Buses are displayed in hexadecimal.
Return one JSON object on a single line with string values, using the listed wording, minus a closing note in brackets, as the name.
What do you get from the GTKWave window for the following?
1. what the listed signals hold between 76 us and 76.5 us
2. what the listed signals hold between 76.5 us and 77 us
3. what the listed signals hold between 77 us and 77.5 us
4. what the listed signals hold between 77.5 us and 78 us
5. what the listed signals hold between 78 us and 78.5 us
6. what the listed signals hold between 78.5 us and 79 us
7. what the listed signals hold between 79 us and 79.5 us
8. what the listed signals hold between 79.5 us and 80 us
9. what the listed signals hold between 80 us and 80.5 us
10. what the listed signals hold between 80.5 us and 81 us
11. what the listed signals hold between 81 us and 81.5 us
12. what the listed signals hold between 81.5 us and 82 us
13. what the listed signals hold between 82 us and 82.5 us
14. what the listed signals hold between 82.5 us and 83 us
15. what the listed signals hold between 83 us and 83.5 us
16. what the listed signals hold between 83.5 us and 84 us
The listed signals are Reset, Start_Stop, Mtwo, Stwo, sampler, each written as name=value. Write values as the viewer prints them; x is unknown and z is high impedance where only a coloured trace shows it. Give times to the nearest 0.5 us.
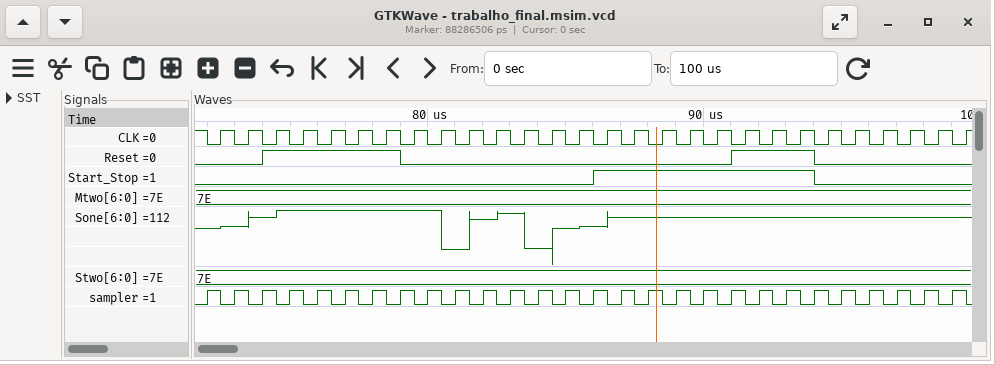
{"what the listed signals hold between 76 us and 76.5 us": "Reset=1, Start_Stop=0, Mtwo=7E, Stwo=7E, sampler=1", "what the listed signals hold between 76.5 us and 77 us": "Reset=1, Start_Stop=0, Mtwo=7E, Stwo=7E, sampler=0", "what the listed signals hold between 77 us and 77.5 us": "Reset=1, Start_Stop=0, Mtwo=7E, Stwo=7E, sampler=1", "what the listed signals hold between 77.5 us and 78 us": "Reset=1, Start_Stop=0, Mtwo=7E, Stwo=7E, sampler=0", "what the listed signals hold between 78 us and 78.5 us": "Reset=1, Start_Stop=0, Mtwo=7E, Stwo=7E, sampler=1", "what the listed signals hold between 78.5 us and 79 us": "Reset=1, Start_Stop=0, Mtwo=7E, Stwo=7E, sampler=0", "what the listed signals hold between 79 us and 79.5 us": "Reset=0, Start_Stop=0, Mtwo=7E, Stwo=7E, sampler=1", "what the listed signals hold between 79.5 us and 80 us": "Reset=0, Start_Stop=0, Mtwo=7E, Stwo=7E, sampler=0", "what the listed signals hold between 80 us and 80.5 us": "Reset=0, Start_Stop=0, Mtwo=7E, Stwo=7E, sampler=1", "what the listed signals hold between 80.5 us and 81 us": "Reset=0, Start_Stop=0, Mtwo=7E, Stwo=7E, sampler=0", "what the listed signals hold between 81 us and 81.5 us": "Reset=0, Start_Stop=0, Mtwo=7E, Stwo=7E, sampler=1", "what the listed signals hold between 81.5 us and 82 us": "Reset=0, Start_Stop=0, Mtwo=7E, Stwo=7E, sampler=0", "what the listed signals hold between 82 us and 82.5 us": "Reset=0, Start_Stop=0, Mtwo=7E, Stwo=7E, sampler=1", "what the listed signals hold between 82.5 us and 83 us": "Reset=0, Start_Stop=0, Mtwo=7E, Stwo=7E, sampler=0", "what the listed signals hold between 83 us and 83.5 us": "Reset=0, Start_Stop=0, Mtwo=7E, Stwo=7E, sampler=1", "what the listed signals hold between 83.5 us and 84 us": "Reset=0, Start_Stop=0, Mtwo=7E, Stwo=7E, sampler=0"}
